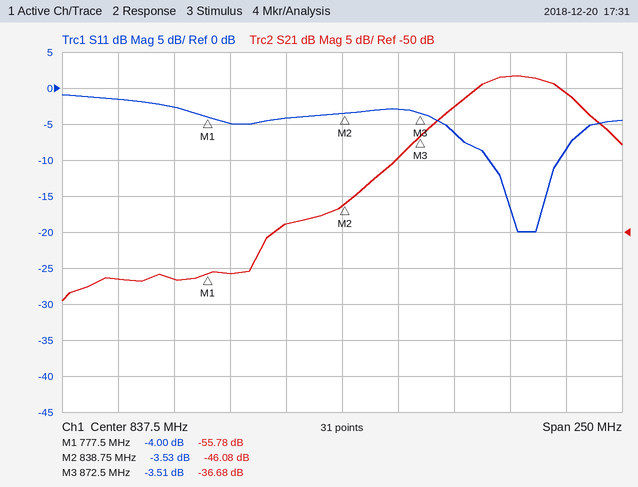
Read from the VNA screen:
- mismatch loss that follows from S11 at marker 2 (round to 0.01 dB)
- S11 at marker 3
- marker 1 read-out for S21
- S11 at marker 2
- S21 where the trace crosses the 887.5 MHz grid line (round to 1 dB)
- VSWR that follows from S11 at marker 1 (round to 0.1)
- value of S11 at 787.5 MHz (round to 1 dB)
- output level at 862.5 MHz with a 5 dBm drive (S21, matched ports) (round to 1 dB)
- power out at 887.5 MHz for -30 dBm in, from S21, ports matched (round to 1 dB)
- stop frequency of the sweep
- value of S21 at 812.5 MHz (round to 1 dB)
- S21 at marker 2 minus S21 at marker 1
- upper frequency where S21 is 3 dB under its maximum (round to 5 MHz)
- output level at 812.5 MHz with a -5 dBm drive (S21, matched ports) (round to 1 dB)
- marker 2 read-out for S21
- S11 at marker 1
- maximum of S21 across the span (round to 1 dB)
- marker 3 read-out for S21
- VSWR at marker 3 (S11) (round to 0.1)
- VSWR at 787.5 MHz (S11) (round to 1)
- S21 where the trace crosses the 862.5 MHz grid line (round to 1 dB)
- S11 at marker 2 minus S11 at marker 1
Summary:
2.55 dB
-3.51 dB
-55.78 dB
-3.53 dB
-33 dB
4.4
-5 dB
-35 dBm
-63 dBm
962.5 MHz
-49 dB
9.70 dB
940 MHz
-54 dBm
-46.08 dB
-4.00 dB
-28 dB
-36.68 dB
5.0
4
-40 dB
0.47 dB
